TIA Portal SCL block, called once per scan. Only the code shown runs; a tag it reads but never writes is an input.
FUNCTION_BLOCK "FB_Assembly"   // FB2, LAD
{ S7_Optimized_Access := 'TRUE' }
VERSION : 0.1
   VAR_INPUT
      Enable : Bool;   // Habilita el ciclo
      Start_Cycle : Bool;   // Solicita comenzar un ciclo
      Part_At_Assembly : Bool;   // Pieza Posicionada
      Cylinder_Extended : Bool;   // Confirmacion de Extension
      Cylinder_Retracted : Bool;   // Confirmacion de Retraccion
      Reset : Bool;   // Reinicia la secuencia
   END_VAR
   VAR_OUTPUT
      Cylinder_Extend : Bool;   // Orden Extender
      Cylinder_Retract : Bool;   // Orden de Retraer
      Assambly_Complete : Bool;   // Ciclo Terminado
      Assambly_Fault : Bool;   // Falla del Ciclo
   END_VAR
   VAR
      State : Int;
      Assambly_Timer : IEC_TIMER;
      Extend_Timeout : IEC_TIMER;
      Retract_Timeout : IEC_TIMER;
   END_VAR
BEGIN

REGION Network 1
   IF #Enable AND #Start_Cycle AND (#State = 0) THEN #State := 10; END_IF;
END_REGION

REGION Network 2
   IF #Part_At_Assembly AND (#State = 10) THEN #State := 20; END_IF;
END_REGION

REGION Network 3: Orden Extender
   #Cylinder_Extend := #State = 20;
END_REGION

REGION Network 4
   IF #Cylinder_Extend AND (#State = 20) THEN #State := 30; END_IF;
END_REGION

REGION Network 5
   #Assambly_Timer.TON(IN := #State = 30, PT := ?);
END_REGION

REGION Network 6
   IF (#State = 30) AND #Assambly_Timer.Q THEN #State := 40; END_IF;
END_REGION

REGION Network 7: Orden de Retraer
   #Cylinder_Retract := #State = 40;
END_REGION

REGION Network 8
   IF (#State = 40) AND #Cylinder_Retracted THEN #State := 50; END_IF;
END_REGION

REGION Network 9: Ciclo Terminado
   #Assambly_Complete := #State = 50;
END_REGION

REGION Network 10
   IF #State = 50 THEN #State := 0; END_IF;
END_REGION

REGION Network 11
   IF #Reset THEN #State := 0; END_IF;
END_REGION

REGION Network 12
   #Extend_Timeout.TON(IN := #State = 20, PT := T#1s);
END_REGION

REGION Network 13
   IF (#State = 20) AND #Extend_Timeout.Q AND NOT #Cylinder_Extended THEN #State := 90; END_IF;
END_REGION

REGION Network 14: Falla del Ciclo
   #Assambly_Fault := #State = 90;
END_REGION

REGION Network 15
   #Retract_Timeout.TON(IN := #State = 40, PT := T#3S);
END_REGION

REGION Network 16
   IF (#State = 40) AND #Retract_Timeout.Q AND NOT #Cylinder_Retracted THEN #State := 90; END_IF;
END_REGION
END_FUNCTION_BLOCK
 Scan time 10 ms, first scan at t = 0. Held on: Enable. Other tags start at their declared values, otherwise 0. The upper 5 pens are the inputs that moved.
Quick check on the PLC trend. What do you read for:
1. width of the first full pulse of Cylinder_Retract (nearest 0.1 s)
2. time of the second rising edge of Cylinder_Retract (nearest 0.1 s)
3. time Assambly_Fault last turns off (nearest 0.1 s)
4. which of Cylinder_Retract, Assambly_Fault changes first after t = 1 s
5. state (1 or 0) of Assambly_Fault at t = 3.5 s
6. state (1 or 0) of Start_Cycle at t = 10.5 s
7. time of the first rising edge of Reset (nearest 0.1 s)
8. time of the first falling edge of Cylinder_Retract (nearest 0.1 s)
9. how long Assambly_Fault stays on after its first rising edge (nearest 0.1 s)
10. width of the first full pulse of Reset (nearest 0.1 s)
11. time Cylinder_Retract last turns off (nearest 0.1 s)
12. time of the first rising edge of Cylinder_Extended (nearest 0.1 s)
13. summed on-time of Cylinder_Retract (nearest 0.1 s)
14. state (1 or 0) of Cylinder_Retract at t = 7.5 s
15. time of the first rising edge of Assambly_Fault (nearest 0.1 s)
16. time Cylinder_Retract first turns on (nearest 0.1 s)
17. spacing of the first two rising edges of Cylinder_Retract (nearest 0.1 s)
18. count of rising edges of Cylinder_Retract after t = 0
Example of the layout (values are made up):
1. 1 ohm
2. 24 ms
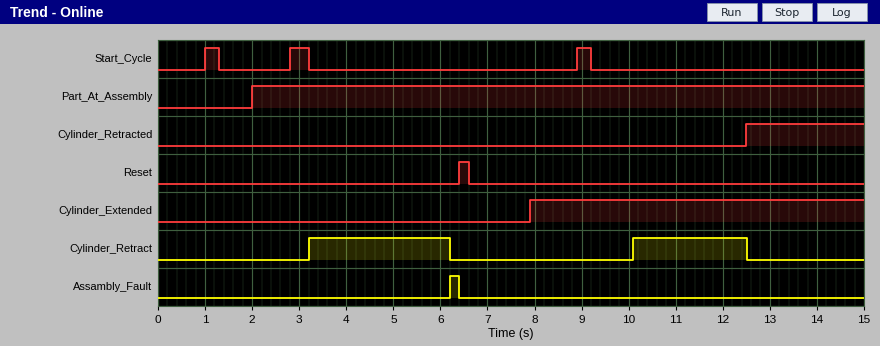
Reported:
1. 3.0 s
2. 10.1 s
3. 6.4 s
4. Cylinder_Retract
5. 0
6. 0
7. 6.4 s
8. 6.2 s
9. 0.2 s
10. 0.2 s
11. 12.5 s
12. 7.9 s
13. 5.4 s
14. 0
15. 6.2 s
16. 3.2 s
17. 6.9 s
18. 2
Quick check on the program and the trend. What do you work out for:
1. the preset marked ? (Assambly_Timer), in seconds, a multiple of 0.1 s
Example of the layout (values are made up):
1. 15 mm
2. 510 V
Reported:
1. 1.2 s
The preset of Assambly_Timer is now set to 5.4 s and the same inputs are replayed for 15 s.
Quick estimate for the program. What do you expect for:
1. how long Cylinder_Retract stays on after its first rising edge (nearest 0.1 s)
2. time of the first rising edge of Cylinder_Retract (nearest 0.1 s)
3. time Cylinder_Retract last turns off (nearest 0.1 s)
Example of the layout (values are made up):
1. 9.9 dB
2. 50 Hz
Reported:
1. 0.0 s
2. 14.3 s
3. 14.3 s
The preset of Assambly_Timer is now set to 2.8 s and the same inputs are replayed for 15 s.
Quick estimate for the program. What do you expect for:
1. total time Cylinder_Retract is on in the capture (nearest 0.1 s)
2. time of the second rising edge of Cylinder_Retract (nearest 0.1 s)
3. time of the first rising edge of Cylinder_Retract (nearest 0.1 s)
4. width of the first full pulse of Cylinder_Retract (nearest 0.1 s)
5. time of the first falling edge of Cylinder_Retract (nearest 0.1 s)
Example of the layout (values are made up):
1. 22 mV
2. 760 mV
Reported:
1. 2.4 s
2. 11.7 s
3. 4.8 s
4. 1.6 s
5. 6.4 s
